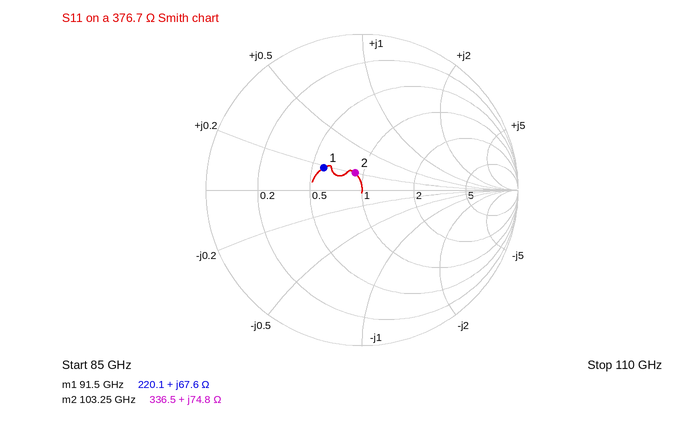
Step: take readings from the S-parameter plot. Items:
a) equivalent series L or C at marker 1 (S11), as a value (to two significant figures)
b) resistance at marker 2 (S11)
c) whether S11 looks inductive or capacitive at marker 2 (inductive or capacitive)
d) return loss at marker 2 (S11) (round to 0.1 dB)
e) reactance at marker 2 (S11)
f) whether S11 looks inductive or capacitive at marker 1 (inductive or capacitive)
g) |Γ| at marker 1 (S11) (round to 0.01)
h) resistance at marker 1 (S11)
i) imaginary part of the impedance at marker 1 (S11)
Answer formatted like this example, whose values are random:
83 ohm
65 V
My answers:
120 pH
336.5 Ω
inductive
18.5 dB
+74.8 Ω
inductive
0.28
220.1 Ω
+67.6 Ω
